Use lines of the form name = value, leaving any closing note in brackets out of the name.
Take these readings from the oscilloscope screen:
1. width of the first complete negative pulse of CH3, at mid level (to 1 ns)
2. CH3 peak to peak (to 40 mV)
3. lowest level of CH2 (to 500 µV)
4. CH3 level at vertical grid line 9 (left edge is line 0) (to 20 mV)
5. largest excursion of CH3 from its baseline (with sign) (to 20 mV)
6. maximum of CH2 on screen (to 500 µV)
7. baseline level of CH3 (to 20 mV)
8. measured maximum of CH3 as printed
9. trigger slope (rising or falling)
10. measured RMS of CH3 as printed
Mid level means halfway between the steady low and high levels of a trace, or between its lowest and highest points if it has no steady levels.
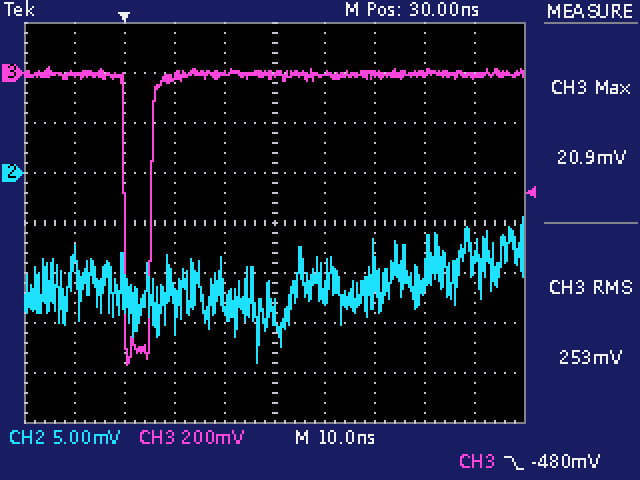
width of the first complete negative pulse of CH3, at mid level = 5 ns
CH3 peak to peak = 1.20 V
lowest level of CH2 = -19.0 mV
CH3 level at vertical grid line 9 (left edge is line 0) = -20 mV
largest excursion of CH3 from its baseline (with sign) = -1.16 V
maximum of CH2 on screen = -4.5 mV
baseline level of CH3 = 0 mV
measured maximum of CH3 as printed = 20.9 mV
trigger slope = falling
measured RMS of CH3 as printed = 253 mV
